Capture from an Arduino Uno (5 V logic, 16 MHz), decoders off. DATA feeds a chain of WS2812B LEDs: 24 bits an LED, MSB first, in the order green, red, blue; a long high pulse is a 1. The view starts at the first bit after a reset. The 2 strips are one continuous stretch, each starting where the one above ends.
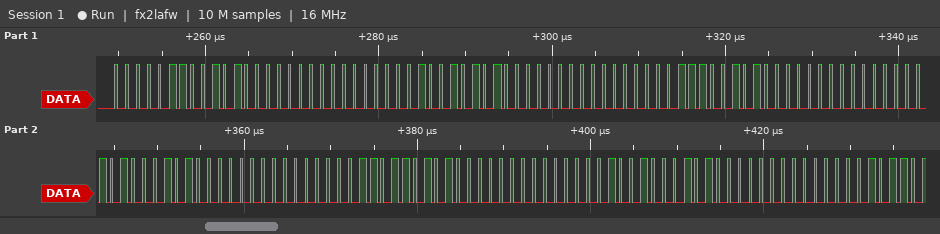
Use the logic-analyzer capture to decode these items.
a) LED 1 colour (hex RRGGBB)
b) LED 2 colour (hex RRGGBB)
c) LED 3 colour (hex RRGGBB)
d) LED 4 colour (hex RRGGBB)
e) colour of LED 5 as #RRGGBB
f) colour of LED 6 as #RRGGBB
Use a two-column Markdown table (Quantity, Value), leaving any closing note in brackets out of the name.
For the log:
| Quantity | Value |
|---|---|
| LED 1 colour | #500600 |
| LED 2 colour | #500900 |
| LED 3 colour | #500E00 |
| LED 4 colour | #501400 |
| colour of LED 5 as #RRGGBB | #501B00 |
| colour of LED 6 as #RRGGBB | #502400 |
